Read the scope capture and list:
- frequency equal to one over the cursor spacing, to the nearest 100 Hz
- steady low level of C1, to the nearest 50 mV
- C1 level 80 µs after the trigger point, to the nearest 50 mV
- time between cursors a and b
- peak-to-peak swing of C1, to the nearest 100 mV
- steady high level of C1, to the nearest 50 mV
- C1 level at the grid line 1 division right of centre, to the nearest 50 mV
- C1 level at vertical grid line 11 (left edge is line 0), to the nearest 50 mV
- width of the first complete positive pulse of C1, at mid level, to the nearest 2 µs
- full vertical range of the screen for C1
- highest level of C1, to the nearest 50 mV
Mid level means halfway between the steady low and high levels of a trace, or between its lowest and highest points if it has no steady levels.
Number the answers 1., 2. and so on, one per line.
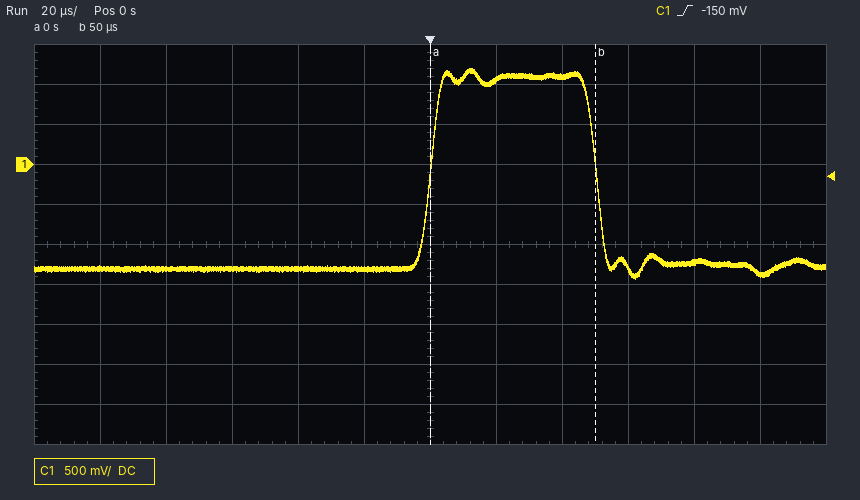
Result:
1. 20.0 kHz
2. -1.30 V
3. -1.20 V
4. 50 µs
5. 2.60 V
6. 1.10 V
7. 1.05 V
8. -1.35 V
9. 50 µs
10. 5 V
11. 1.20 V
